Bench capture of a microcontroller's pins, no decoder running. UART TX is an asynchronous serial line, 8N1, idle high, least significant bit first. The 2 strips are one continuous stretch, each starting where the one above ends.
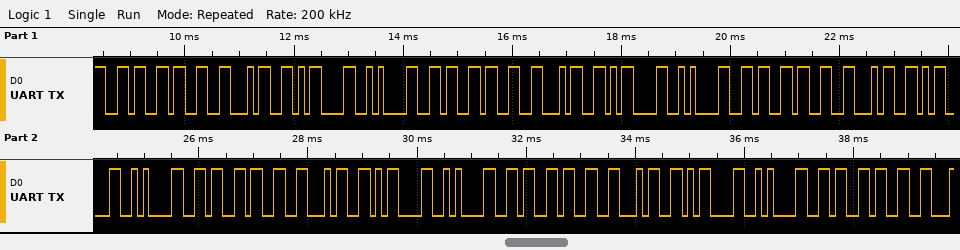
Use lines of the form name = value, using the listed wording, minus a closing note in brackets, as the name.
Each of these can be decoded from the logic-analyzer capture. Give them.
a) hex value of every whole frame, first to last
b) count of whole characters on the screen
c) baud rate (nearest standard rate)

hex value of every whole frame, first to last = 36 33 34 0D 0A 36 33 34 0D 0A 36 33 34 0D 0A 36 33 34 0D 0A 36 33 34 0D 0A 36 33
count of whole characters on the screen = 27
baud rate = 9600 baud
